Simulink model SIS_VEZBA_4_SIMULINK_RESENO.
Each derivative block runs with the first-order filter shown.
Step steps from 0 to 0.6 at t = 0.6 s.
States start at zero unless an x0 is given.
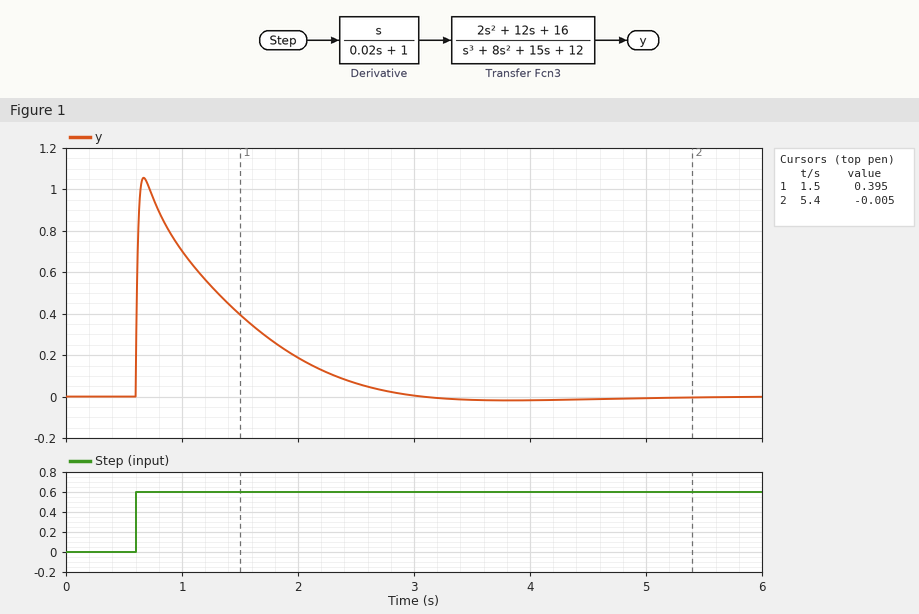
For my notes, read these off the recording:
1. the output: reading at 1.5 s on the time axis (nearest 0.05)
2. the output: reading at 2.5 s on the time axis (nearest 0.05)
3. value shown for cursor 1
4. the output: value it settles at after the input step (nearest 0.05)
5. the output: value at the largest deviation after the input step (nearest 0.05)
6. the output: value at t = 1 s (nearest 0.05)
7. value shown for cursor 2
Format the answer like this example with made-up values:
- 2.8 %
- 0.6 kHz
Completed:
- 0.40
- 0.05
- 0.395
- 0.00
- 1.05
- 0.70
- -0.005
